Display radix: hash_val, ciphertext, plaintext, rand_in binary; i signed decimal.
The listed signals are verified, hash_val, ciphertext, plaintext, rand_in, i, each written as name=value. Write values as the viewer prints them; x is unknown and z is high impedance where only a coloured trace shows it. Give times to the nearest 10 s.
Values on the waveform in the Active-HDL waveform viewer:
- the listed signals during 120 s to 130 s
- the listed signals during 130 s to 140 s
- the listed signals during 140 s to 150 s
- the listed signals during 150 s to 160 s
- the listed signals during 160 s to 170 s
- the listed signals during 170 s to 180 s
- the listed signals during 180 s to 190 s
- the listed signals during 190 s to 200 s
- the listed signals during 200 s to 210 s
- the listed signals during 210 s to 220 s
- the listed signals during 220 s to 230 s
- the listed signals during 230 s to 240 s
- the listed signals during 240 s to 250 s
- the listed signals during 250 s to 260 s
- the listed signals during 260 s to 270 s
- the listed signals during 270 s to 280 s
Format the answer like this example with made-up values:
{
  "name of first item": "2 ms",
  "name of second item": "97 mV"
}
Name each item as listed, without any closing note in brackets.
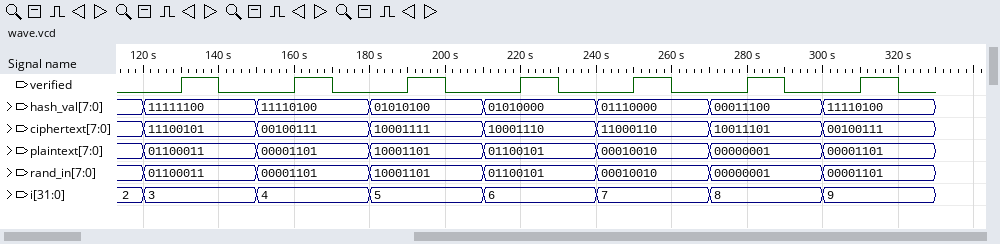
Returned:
{
  "the listed signals during 120 s to 130 s": "verified=0, hash_val=11111100, ciphertext=11100101, plaintext=01100011, rand_in=01100011, i=3",
  "the listed signals during 130 s to 140 s": "verified=1, hash_val=11111100, ciphertext=11100101, plaintext=01100011, rand_in=01100011, i=3",
  "the listed signals during 140 s to 150 s": "verified=0, hash_val=11111100, ciphertext=11100101, plaintext=01100011, rand_in=01100011, i=3",
  "the listed signals during 150 s to 160 s": "verified=0, hash_val=11110100, ciphertext=00100111, plaintext=00001101, rand_in=00001101, i=4",
  "the listed signals during 160 s to 170 s": "verified=1, hash_val=11110100, ciphertext=00100111, plaintext=00001101, rand_in=00001101, i=4",
  "the listed signals during 170 s to 180 s": "verified=0, hash_val=11110100, ciphertext=00100111, plaintext=00001101, rand_in=00001101, i=4",
  "the listed signals during 180 s to 190 s": "verified=0, hash_val=01010100, ciphertext=10001111, plaintext=10001101, rand_in=10001101, i=5",
  "the listed signals during 190 s to 200 s": "verified=1, hash_val=01010100, ciphertext=10001111, plaintext=10001101, rand_in=10001101, i=5",
  "the listed signals during 200 s to 210 s": "verified=0, hash_val=01010100, ciphertext=10001111, plaintext=10001101, rand_in=10001101, i=5",
  "the listed signals during 210 s to 220 s": "verified=0, hash_val=01010000, ciphertext=10001110, plaintext=01100101, rand_in=01100101, i=6",
  "the listed signals during 220 s to 230 s": "verified=1, hash_val=01010000, ciphertext=10001110, plaintext=01100101, rand_in=01100101, i=6",
  "the listed signals during 230 s to 240 s": "verified=0, hash_val=01010000, ciphertext=10001110, plaintext=01100101, rand_in=01100101, i=6",
  "the listed signals during 240 s to 250 s": "verified=0, hash_val=01110000, ciphertext=11000110, plaintext=00010010, rand_in=00010010, i=7",
  "the listed signals during 250 s to 260 s": "verified=1, hash_val=01110000, ciphertext=11000110, plaintext=00010010, rand_in=00010010, i=7",
  "the listed signals during 260 s to 270 s": "verified=0, hash_val=01110000, ciphertext=11000110, plaintext=00010010, rand_in=00010010, i=7",
  "the listed signals during 270 s to 280 s": "verified=0, hash_val=00011100, ciphertext=10011101, plaintext=00000001, rand_in=00000001, i=8"
}
